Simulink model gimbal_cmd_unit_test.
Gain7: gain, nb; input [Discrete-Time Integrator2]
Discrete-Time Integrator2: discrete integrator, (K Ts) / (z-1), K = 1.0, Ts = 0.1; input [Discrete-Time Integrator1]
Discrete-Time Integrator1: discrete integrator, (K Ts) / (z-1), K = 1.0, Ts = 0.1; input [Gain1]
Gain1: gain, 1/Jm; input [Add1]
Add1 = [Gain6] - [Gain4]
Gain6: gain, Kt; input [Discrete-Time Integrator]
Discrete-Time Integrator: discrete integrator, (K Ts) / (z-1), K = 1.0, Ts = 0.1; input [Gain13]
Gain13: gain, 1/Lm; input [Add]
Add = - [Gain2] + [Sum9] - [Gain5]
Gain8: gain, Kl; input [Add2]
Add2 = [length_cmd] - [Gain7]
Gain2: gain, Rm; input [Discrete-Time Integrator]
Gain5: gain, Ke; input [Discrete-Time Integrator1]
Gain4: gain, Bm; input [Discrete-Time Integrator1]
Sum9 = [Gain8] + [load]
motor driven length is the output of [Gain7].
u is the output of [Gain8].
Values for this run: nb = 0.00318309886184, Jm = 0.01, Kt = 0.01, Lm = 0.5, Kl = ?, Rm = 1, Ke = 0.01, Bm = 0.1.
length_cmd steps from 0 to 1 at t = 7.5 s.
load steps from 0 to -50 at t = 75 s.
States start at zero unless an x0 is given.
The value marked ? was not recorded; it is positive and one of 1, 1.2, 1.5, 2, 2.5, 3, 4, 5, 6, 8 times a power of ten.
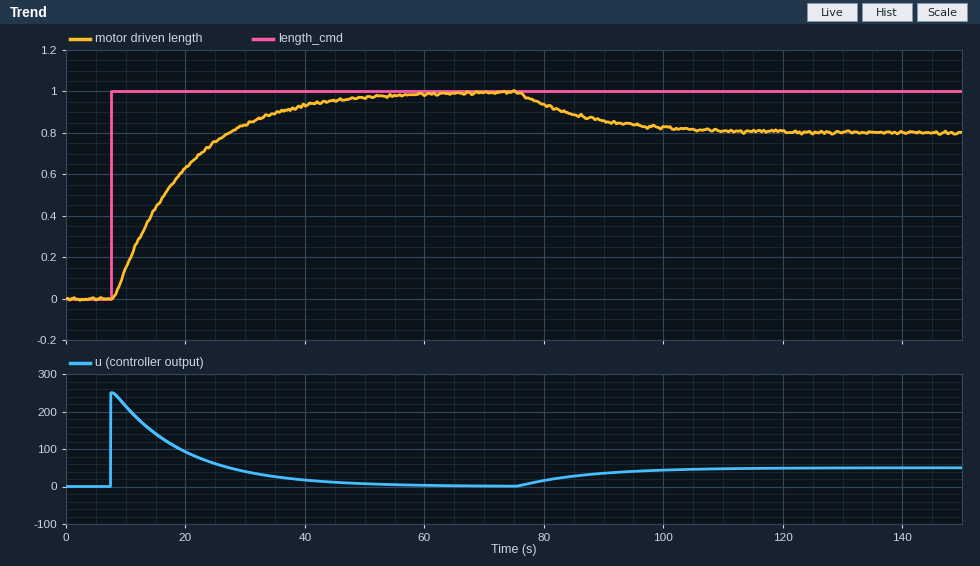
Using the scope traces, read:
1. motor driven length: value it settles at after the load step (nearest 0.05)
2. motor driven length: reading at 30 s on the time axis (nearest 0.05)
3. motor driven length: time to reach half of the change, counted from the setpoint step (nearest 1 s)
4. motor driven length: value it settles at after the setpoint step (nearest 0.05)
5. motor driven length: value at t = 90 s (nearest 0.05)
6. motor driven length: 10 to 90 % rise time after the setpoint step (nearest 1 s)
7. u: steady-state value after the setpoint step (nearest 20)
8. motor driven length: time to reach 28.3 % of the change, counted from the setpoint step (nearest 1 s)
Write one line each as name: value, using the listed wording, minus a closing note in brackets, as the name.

motor driven length: value it settles at after the load step: 0.80
motor driven length: reading at 30 s on the time axis: 0.85
motor driven length: time to reach half of the change, counted from the setpoint step: 9 s
motor driven length: value it settles at after the setpoint step: 1.00
motor driven length: value at t = 90 s: 0.85
motor driven length: 10 to 90 % rise time after the setpoint step: 26 s
u: steady-state value after the setpoint step: 0
motor driven length: time to reach 28.3 % of the change, counted from the setpoint step: 5 s
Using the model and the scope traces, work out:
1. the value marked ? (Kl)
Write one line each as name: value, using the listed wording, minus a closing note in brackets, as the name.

the value marked ?: 250
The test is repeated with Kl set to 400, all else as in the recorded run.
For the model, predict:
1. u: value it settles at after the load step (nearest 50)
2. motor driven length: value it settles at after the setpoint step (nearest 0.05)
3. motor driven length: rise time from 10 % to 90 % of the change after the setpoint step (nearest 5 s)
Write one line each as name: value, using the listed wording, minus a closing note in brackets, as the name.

u: value it settles at after the load step: 50
motor driven length: value it settles at after the setpoint step: 1.00
motor driven length: rise time from 10 % to 90 % of the change after the setpoint step: 15 s
